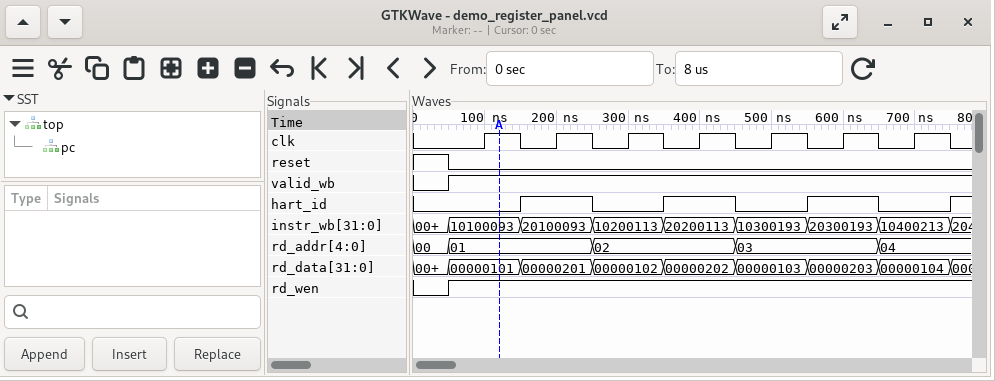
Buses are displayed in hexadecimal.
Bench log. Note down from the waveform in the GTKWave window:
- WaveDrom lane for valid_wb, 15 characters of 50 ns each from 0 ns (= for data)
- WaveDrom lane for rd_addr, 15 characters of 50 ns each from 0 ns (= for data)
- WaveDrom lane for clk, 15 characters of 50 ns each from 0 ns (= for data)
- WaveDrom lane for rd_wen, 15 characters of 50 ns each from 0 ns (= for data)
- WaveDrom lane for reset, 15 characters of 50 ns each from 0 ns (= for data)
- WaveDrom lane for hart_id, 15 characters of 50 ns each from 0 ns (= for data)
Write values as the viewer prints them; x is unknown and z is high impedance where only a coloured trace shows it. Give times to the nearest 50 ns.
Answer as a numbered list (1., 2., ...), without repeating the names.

1. {name: 'valid_wb', wave: '01.............'}
2. {name: 'rd_addr', wave: '==...=...=...=.', data: '00 01 02 03 04'}
3. {name: 'clk', wave: '0.1010101010101'}
4. {name: 'rd_wen', wave: '01.............'}
5. {name: 'reset', wave: '10.............'}
6. {name: 'hart_id', wave: '0..1.0.1.0.1.0.'}
